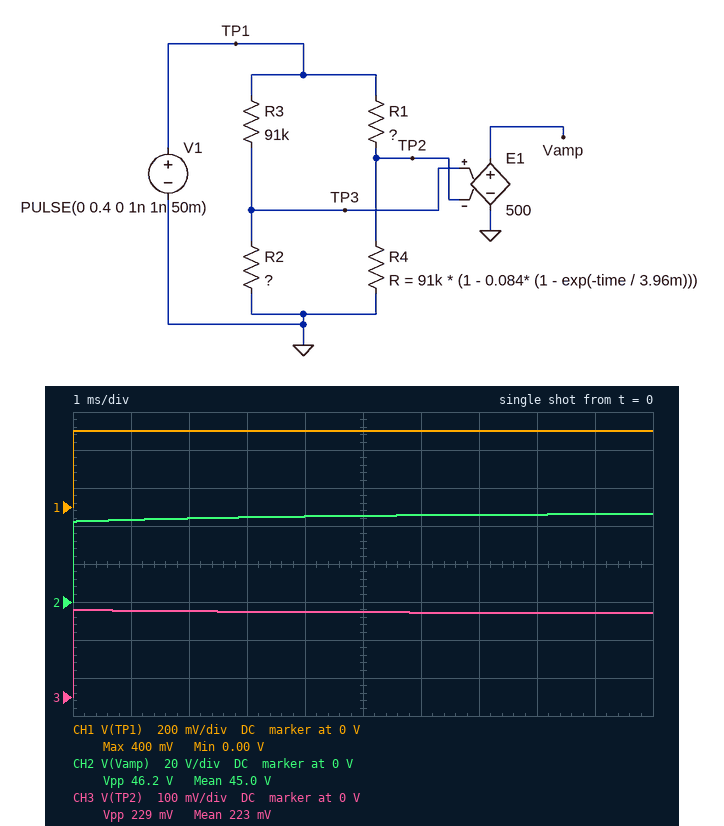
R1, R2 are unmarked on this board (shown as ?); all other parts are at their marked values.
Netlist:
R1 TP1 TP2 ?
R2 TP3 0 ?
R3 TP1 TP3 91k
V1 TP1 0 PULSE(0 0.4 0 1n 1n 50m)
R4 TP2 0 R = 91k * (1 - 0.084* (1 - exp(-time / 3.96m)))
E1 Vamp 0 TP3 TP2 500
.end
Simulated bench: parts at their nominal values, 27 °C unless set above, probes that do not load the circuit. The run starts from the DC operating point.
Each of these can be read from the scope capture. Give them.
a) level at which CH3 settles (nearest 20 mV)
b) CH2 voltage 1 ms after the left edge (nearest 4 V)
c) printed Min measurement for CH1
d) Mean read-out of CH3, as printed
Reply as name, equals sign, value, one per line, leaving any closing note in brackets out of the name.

level at which CH3 settles = 220 mV
CH2 voltage 1 ms after the left edge = 44 V
printed Min measurement for CH1 = 0.00 V
Mean read-out of CH3, as printed = 223 mV
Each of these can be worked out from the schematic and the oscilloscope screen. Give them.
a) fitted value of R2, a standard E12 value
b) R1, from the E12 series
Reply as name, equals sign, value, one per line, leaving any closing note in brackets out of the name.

fitted value of R2, a standard E12 value = 330 kΩ
R1, from the E12 series = 68 kΩ
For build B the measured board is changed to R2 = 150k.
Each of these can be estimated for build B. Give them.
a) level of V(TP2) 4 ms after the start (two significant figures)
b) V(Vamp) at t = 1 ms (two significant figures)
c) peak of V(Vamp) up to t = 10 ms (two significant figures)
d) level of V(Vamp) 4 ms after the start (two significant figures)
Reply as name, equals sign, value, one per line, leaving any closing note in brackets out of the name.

level of V(TP2) 4 ms after the start = 220 mV
V(Vamp) at t = 1 ms = 11 V
peak of V(Vamp) up to t = 10 ms = 14 V
level of V(Vamp) 4 ms after the start = 13 V
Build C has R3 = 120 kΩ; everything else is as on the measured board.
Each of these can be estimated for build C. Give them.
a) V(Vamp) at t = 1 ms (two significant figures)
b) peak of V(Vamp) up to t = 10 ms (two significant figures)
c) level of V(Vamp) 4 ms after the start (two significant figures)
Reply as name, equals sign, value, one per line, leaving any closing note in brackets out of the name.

V(Vamp) at t = 1 ms = 33 V
peak of V(Vamp) up to t = 10 ms = 36 V
level of V(Vamp) 4 ms after the start = 35 V
